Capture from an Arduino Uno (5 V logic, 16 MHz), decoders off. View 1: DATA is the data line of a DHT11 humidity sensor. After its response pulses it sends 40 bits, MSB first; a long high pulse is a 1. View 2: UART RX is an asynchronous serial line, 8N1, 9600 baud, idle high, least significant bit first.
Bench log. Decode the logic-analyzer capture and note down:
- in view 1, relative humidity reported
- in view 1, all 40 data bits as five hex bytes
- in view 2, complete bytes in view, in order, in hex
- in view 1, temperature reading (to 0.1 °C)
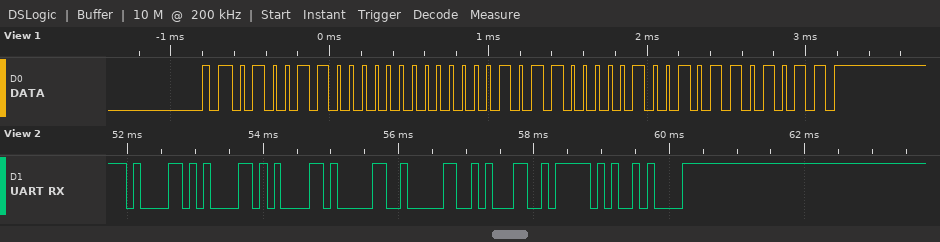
76 %
4C 00 16 09 6B
61 61 61 30 30 31 5F 0A
22.9 °C
